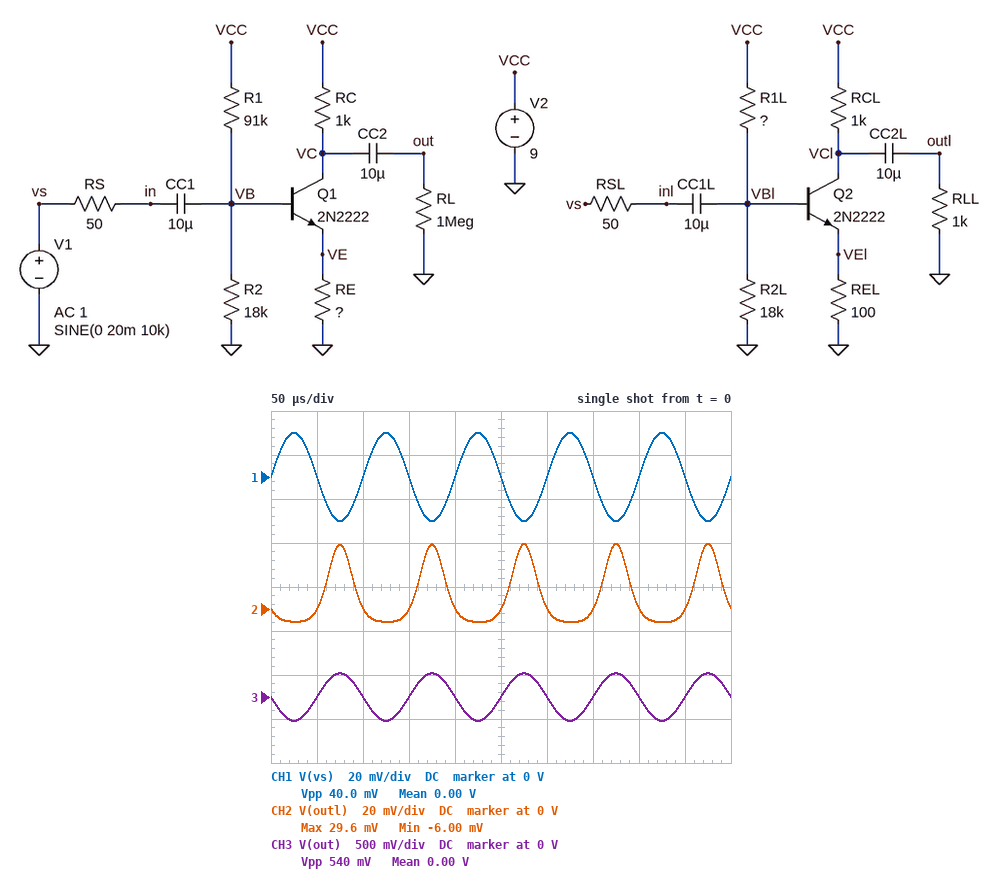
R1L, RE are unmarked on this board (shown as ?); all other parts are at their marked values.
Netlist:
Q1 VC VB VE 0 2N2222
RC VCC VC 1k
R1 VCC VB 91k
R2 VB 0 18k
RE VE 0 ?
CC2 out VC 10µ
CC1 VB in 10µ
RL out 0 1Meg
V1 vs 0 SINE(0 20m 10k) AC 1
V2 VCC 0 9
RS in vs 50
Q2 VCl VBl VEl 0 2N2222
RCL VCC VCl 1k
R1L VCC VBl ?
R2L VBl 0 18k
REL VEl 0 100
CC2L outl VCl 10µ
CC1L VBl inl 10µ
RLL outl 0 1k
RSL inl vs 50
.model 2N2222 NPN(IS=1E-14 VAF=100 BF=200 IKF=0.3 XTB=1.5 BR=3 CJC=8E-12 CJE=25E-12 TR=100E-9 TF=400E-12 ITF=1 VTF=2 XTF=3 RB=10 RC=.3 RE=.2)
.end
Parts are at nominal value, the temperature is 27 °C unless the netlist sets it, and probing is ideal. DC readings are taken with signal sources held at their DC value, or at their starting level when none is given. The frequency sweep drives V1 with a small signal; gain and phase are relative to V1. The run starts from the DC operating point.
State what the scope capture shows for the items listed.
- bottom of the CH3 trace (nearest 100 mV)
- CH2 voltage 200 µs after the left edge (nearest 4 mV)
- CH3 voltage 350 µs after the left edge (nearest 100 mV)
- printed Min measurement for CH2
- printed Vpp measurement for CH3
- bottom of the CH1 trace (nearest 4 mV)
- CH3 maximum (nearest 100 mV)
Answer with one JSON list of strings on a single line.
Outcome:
["-300 mV", "0 V", "0 V", "-6.00 mV", "540 mV", "-20 mV", "300 mV"]
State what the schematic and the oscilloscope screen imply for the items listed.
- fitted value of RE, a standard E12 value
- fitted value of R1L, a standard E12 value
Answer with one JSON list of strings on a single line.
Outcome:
["68 Ω", "33 kΩ"]
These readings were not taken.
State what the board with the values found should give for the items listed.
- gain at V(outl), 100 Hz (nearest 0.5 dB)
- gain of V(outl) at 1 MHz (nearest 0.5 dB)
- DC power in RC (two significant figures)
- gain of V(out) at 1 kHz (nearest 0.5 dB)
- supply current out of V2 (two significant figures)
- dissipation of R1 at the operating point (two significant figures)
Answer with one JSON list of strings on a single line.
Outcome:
["-6.5 dB", "-4.5 dB", "30 mW", "22.5 dB", "14 mA", "690 µW"]
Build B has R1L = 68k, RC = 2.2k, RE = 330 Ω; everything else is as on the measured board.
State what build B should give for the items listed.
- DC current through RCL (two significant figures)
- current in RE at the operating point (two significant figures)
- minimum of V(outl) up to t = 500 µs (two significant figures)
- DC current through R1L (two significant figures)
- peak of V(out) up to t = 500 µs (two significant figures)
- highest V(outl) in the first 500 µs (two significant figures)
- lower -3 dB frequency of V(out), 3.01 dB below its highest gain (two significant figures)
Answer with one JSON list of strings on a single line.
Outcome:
["6.8 mA", "2.0 mA", "-95 mV", "110 µA", "130 mV", "95 mV", "1.3 Hz"]
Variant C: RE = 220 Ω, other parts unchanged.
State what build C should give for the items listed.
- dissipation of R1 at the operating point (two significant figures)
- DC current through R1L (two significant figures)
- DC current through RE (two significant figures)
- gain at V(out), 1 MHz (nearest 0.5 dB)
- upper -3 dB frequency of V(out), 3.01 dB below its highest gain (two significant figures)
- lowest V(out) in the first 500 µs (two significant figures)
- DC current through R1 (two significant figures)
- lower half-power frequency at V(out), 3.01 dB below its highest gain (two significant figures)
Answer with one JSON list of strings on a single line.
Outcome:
["650 µW", "230 µA", "2.8 mA", "12.5 dB", "30 MHz", "-86 mV", "85 µA", "1.4 Hz"]
